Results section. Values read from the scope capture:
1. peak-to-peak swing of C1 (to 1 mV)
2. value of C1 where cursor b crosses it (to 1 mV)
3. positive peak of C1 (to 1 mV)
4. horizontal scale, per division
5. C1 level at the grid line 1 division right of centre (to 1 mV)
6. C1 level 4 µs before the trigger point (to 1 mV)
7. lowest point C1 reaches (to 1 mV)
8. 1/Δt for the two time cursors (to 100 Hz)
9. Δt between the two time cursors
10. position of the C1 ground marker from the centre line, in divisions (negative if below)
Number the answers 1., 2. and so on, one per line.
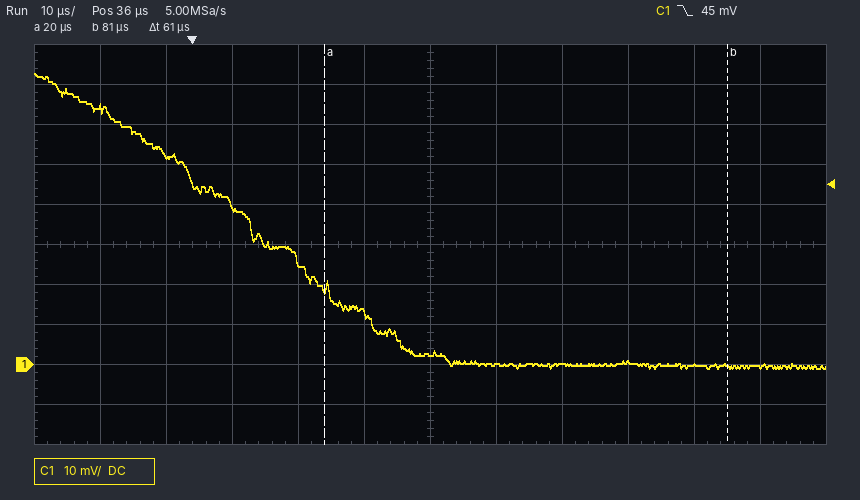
1. 74 mV
2. 0 mV
3. 73 mV
4. 10 µs
5. 0 mV
6. 52 mV
7. -1 mV
8. 16.4 kHz
9. 61 µs
10. -3.0 div
